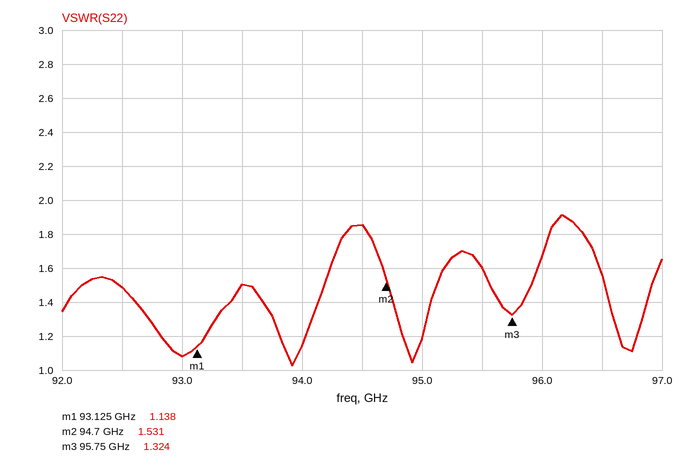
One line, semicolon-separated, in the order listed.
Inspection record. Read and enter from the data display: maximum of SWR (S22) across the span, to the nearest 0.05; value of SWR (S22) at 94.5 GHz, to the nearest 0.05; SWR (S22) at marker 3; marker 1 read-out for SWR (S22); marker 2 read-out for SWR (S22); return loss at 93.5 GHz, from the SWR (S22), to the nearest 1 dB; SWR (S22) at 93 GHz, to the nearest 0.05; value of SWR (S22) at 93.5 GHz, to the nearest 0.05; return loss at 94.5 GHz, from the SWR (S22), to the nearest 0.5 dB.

1.90; 1.85; 1.324; 1.138; 1.531; 14 dB; 1.10; 1.50; 10.5 dB
